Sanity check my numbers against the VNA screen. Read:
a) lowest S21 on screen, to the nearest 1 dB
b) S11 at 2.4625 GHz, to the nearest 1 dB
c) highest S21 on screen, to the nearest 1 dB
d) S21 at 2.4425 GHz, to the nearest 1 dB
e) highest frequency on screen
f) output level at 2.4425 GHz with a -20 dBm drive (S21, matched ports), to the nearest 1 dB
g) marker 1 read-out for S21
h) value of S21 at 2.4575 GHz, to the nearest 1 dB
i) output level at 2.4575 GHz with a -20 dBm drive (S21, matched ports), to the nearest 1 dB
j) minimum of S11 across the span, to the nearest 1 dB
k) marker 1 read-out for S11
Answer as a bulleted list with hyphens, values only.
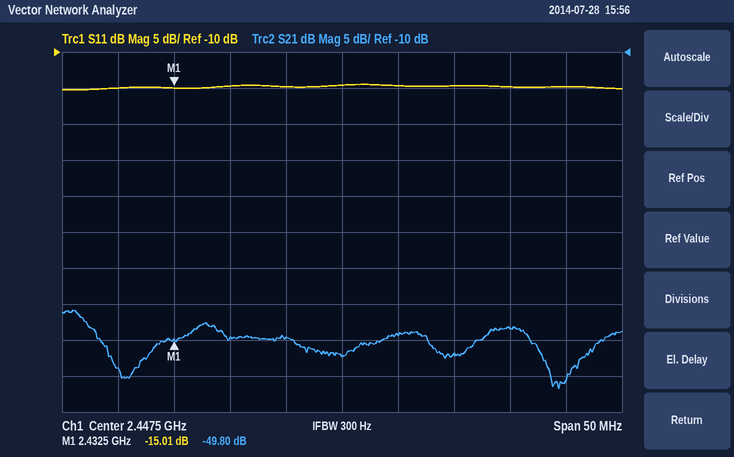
- -57 dB
- -15 dB
- -46 dB
- -50 dB
- 2.4725 GHz
- -70 dBm
- -49.80 dB
- -52 dB
- -72 dBm
- -15 dB
- -15.01 dB
